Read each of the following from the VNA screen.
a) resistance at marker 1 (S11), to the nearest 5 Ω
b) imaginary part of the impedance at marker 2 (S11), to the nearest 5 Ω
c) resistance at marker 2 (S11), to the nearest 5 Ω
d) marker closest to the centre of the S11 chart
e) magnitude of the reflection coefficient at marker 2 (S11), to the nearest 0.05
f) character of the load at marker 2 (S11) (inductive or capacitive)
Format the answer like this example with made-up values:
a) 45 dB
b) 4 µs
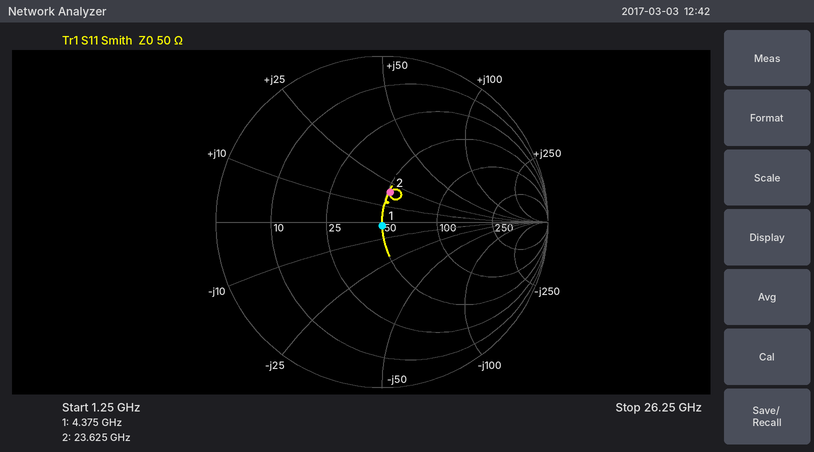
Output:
a) 50 Ω
b) +20 Ω
c) 50 Ω
d) marker 1
e) 0.20
f) inductive
